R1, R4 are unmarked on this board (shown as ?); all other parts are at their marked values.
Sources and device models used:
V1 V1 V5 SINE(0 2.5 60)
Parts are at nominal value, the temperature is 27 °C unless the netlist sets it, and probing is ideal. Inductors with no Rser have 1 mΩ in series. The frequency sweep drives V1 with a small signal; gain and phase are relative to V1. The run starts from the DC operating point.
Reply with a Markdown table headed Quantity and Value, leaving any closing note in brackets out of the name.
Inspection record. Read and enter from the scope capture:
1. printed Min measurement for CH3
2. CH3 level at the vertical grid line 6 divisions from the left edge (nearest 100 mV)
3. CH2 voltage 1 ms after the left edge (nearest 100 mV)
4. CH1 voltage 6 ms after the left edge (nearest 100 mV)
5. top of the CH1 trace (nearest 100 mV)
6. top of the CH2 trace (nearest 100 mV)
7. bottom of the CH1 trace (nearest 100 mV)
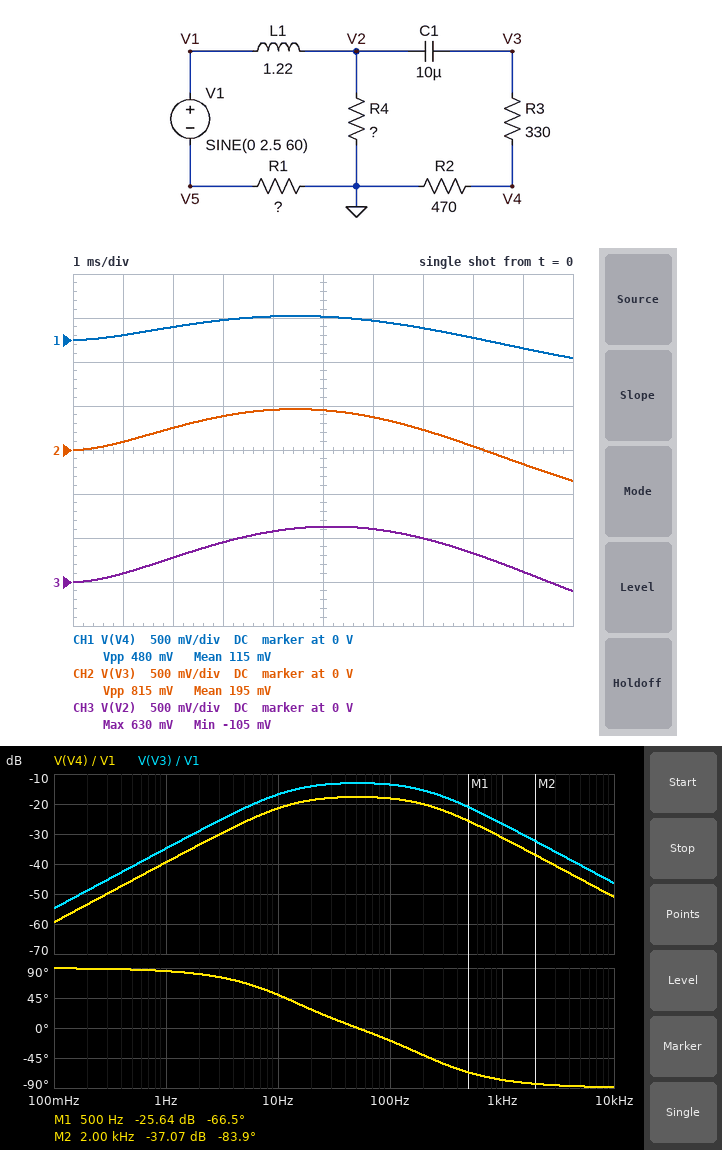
| Quantity | Value |
|---|---|
| printed Min measurement for CH3 | -105 mV |
| CH3 level at the vertical grid line 6 divisions from the left edge | 600 mV |
| CH2 voltage 1 ms after the left edge | 100 mV |
| CH1 voltage 6 ms after the left edge | 200 mV |
| top of the CH1 trace | 300 mV |
| top of the CH2 trace | 500 mV |
| bottom of the CH1 trace | -200 mV |
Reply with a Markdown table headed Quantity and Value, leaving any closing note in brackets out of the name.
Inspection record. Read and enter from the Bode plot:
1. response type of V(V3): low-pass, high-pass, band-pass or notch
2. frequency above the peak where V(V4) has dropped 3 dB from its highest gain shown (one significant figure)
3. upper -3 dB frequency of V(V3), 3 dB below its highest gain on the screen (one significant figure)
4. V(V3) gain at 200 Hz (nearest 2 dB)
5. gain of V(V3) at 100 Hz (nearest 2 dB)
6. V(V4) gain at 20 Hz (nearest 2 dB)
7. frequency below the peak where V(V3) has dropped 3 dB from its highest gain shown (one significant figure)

| Quantity | Value |
|---|---|
| response type of V(V3): low-pass, high-pass, band-pass or notch | band-pass |
| frequency above the peak where V(V4) has dropped 3 dB from its highest gain shown | 200 Hz |
| upper -3 dB frequency of V(V3), 3 dB below its highest gain on the screen | 200 Hz |
| V(V3) gain at 200 Hz | -16 dB |
| gain of V(V3) at 100 Hz | -14 dB |
| V(V4) gain at 20 Hz | -18 dB |
| frequency below the peak where V(V3) has dropped 3 dB from its highest gain shown | 10 Hz |
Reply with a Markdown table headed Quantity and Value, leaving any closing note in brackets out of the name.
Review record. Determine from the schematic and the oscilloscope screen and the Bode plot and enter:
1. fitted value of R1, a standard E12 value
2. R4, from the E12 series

| Quantity | Value |
|---|---|
| fitted value of R1, a standard E12 value | 1.2 kΩ |
| R4, from the E12 series | 680 Ω |
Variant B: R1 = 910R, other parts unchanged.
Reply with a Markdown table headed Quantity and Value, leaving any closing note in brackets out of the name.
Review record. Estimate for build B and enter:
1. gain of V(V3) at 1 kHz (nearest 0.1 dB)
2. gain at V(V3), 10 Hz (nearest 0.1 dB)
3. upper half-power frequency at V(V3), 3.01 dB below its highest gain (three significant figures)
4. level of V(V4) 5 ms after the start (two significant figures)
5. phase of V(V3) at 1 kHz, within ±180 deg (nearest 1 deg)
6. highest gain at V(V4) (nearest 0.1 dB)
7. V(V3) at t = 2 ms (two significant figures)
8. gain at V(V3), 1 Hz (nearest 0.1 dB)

| Quantity | Value |
|---|---|
| gain of V(V3) at 1 kHz | -26.5 dB |
| gain at V(V3), 10 Hz | -15.2 dB |
| upper half-power frequency at V(V3), 3.01 dB below its highest gain | 189 Hz |
| level of V(V4) 5 ms after the start | 320 mV |
| phase of V(V3) at 1 kHz, within ±180 deg | -80 deg |
| highest gain at V(V4) | -16.0 dB |
| V(V3) at t = 2 ms | 280 mV |
| gain at V(V3), 1 Hz | -33.4 dB |
